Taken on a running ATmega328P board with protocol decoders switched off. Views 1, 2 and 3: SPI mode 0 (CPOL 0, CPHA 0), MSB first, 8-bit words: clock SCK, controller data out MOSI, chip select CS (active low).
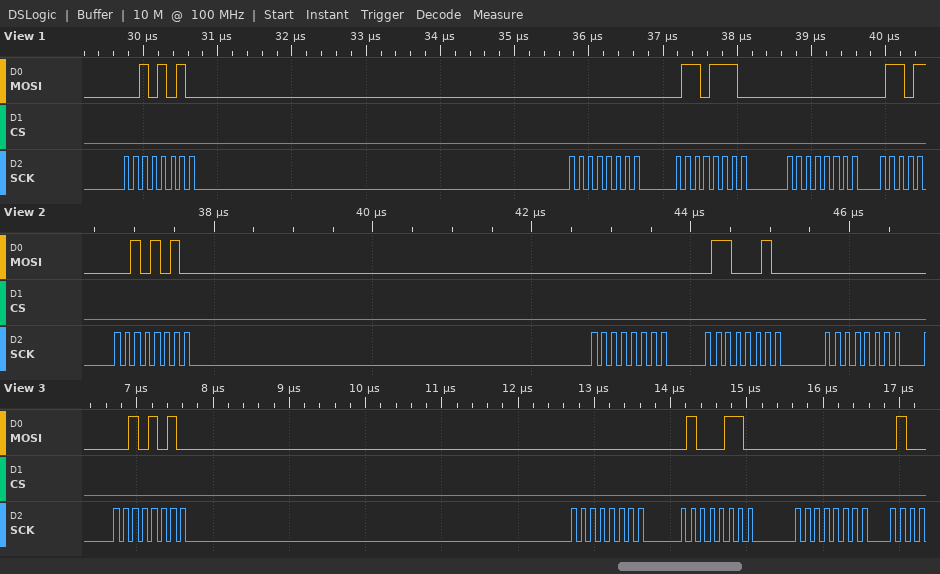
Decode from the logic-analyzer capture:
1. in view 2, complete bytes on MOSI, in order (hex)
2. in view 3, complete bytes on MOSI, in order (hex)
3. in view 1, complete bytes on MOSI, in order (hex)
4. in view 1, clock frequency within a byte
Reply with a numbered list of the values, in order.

1. 2A 00 62 00
2. 2A 00 46 00
3. 2A 00 6E 00
4. 8 MHz
